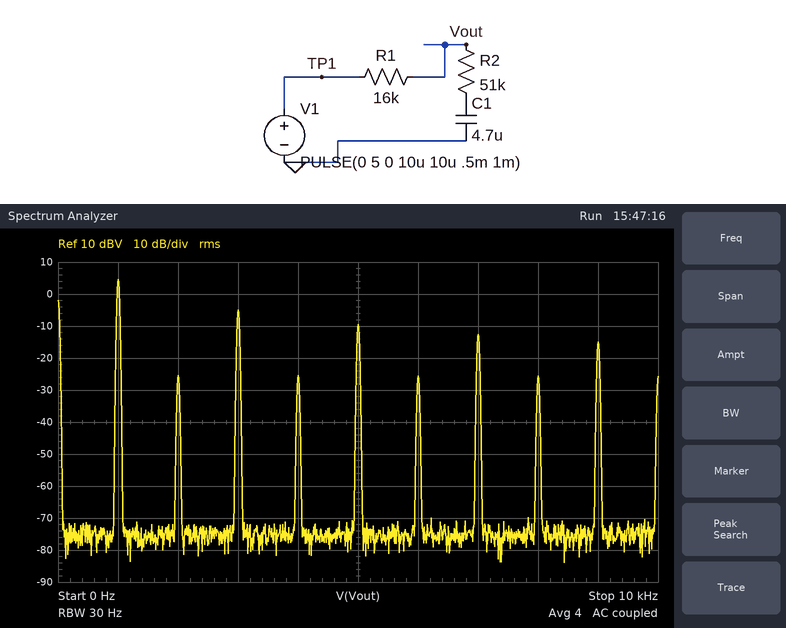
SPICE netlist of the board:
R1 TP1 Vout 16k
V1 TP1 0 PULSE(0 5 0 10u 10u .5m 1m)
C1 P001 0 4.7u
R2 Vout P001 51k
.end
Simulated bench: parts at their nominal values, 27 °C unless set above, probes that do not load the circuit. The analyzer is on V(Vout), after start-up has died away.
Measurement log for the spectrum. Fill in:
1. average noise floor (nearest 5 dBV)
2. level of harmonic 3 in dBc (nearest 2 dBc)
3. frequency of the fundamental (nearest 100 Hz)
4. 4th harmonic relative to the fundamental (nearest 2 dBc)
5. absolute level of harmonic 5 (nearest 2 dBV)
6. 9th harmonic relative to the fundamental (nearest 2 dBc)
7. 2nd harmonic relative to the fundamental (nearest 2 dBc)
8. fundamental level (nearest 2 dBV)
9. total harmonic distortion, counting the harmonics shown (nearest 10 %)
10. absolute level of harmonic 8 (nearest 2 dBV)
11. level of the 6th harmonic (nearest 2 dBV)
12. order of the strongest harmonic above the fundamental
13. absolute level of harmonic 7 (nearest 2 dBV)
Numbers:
-75 dBV
-10 dBc
1.0 kHz
-30 dBc
-10 dBV
-20 dBc
-30 dBc
4 dBV
40 %
-26 dBV
-26 dBV
3
-12 dBV
